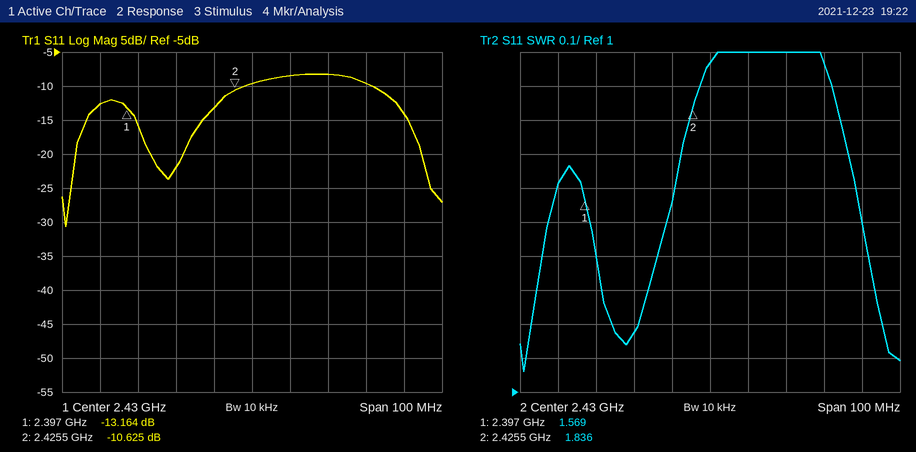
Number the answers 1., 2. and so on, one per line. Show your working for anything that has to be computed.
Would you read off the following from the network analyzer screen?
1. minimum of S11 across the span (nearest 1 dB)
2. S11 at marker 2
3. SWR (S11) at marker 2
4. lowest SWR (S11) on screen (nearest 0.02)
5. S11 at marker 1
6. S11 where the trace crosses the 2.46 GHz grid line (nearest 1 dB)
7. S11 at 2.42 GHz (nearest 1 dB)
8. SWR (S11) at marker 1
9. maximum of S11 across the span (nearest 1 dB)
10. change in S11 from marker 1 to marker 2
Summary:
1. -31 dB
2. -10.625 dB
3. 1.836
4. 1.06
5. -13.164 dB
6. -10 dB
7. -13 dB
8. 1.569
9. -8 dB
10. -10.625 − (-13.164) = 2.539 dB
